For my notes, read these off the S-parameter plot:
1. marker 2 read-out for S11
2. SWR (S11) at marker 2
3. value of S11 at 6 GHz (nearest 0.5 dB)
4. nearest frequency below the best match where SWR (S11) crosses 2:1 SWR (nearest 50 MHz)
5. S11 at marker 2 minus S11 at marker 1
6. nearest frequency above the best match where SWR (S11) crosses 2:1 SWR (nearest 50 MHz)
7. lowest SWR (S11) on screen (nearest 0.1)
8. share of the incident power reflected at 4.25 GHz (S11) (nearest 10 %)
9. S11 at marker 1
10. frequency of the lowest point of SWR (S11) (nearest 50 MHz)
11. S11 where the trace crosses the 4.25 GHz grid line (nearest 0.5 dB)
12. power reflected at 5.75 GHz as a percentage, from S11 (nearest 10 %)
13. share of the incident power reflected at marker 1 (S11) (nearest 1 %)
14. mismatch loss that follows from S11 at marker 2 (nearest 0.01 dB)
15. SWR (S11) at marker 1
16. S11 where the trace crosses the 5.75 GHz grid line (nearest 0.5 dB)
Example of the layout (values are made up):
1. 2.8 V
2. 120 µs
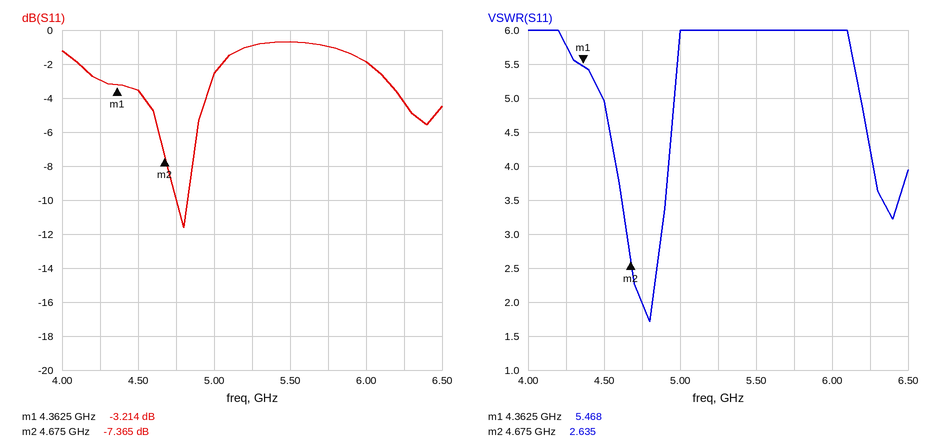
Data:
1. -7.365 dB
2. 2.635
3. -2.0 dB
4. 4.75 GHz
5. -4.151 dB
6. 4.80 GHz
7. 1.7
8. 50 %
9. -3.214 dB
10. 4.80 GHz
11. -3.0 dB
12. 80 %
13. 48 %
14. 0.88 dB
15. 5.468
16. -1.0 dB
